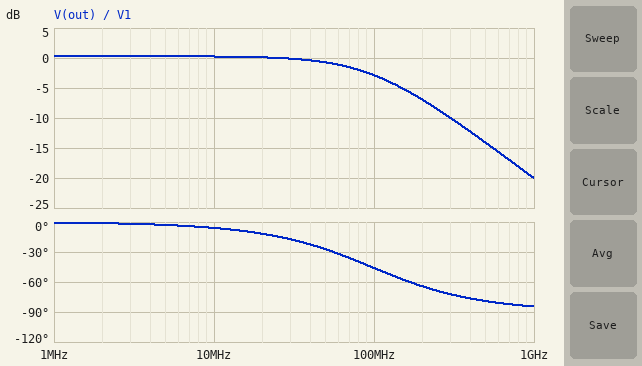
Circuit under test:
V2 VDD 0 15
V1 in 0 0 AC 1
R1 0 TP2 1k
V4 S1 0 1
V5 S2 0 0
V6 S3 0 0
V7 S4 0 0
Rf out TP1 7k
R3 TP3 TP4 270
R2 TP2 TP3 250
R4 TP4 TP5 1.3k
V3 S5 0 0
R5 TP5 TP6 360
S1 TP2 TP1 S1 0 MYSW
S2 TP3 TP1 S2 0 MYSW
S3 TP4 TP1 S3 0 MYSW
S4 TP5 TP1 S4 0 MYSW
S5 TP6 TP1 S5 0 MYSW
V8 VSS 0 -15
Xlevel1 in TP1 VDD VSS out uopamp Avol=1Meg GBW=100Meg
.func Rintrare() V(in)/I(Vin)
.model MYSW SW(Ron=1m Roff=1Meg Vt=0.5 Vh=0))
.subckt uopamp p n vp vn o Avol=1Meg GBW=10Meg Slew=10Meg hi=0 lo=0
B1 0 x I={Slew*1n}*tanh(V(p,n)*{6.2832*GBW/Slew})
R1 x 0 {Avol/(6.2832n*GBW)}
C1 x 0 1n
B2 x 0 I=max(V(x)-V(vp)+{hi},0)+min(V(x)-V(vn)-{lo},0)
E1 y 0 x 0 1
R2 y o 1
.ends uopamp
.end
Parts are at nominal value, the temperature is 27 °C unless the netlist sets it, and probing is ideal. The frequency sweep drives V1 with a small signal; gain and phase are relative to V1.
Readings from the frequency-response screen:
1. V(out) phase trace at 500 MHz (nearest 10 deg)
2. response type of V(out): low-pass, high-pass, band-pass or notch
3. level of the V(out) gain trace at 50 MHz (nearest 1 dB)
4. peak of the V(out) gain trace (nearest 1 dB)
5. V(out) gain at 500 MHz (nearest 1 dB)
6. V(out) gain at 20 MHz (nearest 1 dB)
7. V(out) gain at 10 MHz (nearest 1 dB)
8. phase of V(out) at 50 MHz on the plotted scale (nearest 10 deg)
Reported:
-80 deg
low-pass
-1 dB
0 dB
-14 dB
0 dB
0 dB
-30 deg
